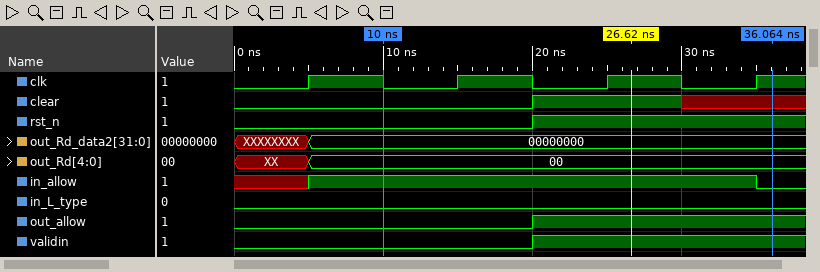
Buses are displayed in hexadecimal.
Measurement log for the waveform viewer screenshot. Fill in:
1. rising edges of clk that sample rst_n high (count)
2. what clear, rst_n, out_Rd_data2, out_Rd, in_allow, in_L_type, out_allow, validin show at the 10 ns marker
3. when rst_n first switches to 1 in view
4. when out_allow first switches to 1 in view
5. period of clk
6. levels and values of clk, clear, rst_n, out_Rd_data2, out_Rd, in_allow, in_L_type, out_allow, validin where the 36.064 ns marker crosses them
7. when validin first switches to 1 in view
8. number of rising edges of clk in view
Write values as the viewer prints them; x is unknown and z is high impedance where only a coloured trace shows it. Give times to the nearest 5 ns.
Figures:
2
clear=0, rst_n=0, out_Rd_data2=00000000, out_Rd=00, in_allow=1, in_L_type=0, out_allow=0, validin=0
20 ns
20 ns
10 ns
clk=1, clear=x, rst_n=1, out_Rd_data2=00000000, out_Rd=00, in_allow=0, in_L_type=0, out_allow=1, validin=1
20 ns
4
